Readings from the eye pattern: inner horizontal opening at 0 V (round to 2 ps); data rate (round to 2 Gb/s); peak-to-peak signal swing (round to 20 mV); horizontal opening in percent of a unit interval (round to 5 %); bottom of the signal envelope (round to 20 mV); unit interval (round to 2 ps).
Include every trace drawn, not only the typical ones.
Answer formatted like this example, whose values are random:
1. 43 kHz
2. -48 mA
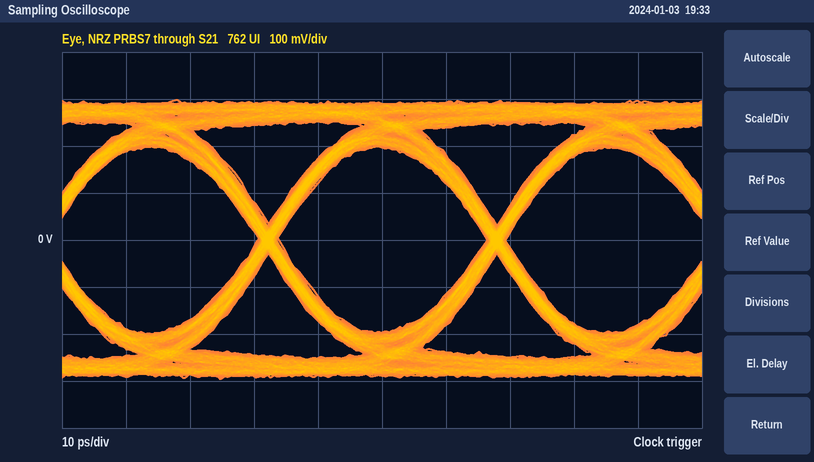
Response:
1. 32 ps
2. 28 Gb/s
3. 600 mV
4. 90 %
5. -300 mV
6. 36 ps
